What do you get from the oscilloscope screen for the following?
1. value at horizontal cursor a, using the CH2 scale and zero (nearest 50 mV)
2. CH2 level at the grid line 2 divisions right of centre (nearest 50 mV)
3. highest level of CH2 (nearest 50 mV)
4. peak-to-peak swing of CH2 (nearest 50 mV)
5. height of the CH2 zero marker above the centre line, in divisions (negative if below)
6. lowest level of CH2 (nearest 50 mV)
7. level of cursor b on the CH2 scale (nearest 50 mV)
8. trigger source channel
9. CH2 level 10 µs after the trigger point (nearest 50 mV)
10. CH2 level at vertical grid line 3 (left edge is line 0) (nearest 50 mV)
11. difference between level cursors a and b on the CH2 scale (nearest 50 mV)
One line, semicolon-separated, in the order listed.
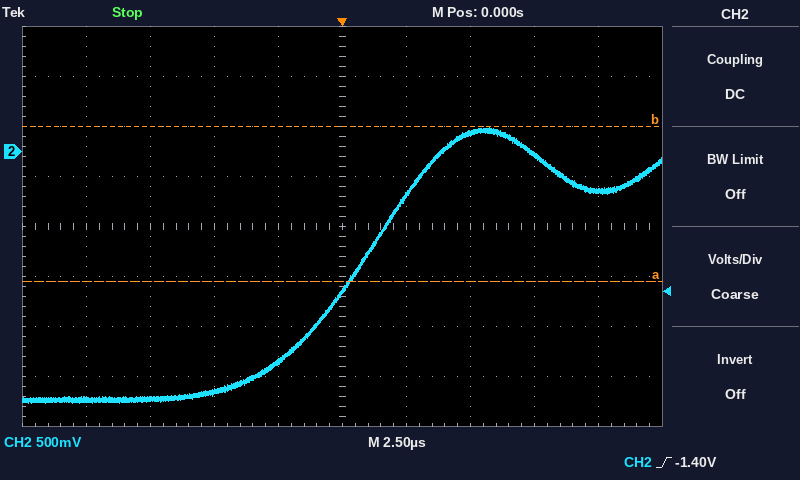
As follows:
-1.30 V; 200 mV; 250 mV; 2.75 V; +1.5 div; -2.50 V; 250 mV; CH2; -400 mV; -2.40 V; 1.55 V
